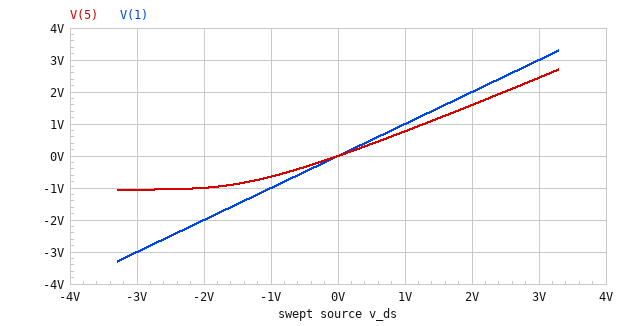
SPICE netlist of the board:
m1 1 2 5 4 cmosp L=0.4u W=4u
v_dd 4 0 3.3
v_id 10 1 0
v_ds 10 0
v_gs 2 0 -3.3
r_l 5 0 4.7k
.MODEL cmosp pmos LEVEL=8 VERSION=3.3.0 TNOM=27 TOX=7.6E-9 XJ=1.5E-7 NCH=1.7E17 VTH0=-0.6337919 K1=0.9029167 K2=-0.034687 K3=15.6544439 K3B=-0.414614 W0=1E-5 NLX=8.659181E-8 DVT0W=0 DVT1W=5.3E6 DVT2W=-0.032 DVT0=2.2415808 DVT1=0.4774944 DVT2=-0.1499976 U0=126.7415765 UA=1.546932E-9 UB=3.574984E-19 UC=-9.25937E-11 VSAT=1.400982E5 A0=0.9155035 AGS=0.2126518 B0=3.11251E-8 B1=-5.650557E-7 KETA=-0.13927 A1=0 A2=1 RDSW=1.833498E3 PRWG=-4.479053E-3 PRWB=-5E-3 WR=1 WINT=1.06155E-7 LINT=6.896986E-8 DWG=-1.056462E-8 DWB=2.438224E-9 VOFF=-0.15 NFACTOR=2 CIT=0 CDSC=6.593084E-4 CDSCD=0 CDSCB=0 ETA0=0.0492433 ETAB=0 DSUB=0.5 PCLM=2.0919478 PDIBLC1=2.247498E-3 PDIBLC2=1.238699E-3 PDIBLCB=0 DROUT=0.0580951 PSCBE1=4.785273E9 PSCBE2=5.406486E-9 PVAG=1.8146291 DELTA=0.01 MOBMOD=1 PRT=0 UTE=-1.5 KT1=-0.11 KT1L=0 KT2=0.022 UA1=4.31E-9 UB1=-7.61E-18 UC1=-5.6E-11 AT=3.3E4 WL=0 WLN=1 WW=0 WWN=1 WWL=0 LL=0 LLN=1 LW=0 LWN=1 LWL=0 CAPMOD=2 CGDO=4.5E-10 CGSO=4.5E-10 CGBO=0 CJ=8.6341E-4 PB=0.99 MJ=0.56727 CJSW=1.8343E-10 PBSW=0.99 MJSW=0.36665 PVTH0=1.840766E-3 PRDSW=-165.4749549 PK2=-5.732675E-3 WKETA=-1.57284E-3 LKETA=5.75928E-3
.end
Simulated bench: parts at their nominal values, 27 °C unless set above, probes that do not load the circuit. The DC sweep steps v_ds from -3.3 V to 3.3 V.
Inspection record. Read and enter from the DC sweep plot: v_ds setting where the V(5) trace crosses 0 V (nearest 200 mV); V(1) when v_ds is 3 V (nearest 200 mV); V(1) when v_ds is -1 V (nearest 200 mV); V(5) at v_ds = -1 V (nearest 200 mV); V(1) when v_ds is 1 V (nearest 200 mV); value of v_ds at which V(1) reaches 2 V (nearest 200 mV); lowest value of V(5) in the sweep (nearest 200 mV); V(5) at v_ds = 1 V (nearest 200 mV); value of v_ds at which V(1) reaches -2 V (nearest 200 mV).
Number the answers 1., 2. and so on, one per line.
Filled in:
1. 0 V
2. 3.0 V
3. -1.0 V
4. -600 mV
5. 1.0 V
6. 2.0 V
7. -1.0 V
8. 800 mV
9. -2.0 V
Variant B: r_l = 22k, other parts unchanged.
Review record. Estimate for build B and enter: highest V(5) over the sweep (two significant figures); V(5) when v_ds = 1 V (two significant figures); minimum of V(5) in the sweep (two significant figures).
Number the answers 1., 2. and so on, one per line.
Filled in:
1. 3.2 V
2. 940 mV
3. -1.5 V
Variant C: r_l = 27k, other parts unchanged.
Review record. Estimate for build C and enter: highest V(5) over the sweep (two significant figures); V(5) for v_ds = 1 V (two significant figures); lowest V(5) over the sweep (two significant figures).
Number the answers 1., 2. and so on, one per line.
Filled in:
1. 3.2 V
2. 950 mV
3. -1.5 V
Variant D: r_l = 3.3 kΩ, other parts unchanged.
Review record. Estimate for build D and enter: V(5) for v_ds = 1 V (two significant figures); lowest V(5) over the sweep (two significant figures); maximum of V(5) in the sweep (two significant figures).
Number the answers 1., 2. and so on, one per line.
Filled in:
1. 700 mV
2. -940 mV
3. 2.5 V
